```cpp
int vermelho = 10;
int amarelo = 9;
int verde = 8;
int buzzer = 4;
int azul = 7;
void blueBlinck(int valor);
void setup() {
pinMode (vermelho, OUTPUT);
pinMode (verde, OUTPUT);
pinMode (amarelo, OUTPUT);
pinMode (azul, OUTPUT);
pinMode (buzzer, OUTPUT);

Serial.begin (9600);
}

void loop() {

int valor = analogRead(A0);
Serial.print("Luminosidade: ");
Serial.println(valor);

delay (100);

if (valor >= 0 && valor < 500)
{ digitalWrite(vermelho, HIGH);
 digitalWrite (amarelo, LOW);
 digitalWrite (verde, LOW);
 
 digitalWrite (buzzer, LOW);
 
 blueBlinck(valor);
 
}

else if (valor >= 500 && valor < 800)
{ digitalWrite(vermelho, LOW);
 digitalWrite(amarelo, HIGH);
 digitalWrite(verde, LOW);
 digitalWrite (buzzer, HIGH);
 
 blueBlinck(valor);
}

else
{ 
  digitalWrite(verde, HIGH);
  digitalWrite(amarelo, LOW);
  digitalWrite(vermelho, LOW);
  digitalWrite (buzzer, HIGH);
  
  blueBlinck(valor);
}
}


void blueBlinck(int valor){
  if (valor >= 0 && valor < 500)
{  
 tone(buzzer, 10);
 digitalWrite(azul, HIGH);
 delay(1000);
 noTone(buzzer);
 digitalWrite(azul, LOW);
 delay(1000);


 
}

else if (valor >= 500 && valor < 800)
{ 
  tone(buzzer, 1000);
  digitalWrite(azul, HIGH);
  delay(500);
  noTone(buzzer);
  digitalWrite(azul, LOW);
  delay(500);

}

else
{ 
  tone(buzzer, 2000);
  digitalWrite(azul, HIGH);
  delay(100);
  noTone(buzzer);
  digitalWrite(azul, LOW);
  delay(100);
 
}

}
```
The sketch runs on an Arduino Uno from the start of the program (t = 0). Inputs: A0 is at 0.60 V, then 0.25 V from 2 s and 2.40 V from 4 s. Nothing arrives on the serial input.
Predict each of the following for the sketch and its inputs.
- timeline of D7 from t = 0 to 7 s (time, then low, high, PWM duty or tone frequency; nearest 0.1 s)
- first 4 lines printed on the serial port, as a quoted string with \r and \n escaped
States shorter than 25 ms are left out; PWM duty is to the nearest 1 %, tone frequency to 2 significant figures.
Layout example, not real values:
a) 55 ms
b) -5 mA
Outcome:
a) 0 s low; 0.1 s high; 1.1 s low; 2.2 s high; 3.2 s low; 4.3 s high; 5.3 s low; 6.4 s high
b) "Luminosidade: 122\r\nLuminosidade: 51\r\nLuminosidade: 491\r\nLuminosidade: 491\r\n"
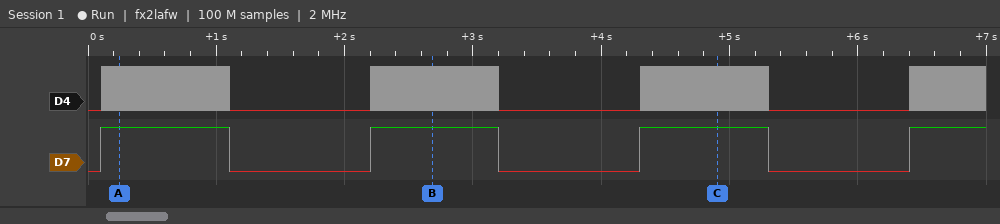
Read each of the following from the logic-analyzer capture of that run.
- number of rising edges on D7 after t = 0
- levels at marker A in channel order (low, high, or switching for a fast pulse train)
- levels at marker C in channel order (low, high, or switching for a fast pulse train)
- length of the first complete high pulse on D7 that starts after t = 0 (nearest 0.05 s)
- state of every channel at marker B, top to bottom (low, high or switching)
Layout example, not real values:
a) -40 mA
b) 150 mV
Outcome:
a) 4
b) D4 switching, D7 high
c) D4 switching, D7 high
d) 1.00 s
e) D4 switching, D7 high
